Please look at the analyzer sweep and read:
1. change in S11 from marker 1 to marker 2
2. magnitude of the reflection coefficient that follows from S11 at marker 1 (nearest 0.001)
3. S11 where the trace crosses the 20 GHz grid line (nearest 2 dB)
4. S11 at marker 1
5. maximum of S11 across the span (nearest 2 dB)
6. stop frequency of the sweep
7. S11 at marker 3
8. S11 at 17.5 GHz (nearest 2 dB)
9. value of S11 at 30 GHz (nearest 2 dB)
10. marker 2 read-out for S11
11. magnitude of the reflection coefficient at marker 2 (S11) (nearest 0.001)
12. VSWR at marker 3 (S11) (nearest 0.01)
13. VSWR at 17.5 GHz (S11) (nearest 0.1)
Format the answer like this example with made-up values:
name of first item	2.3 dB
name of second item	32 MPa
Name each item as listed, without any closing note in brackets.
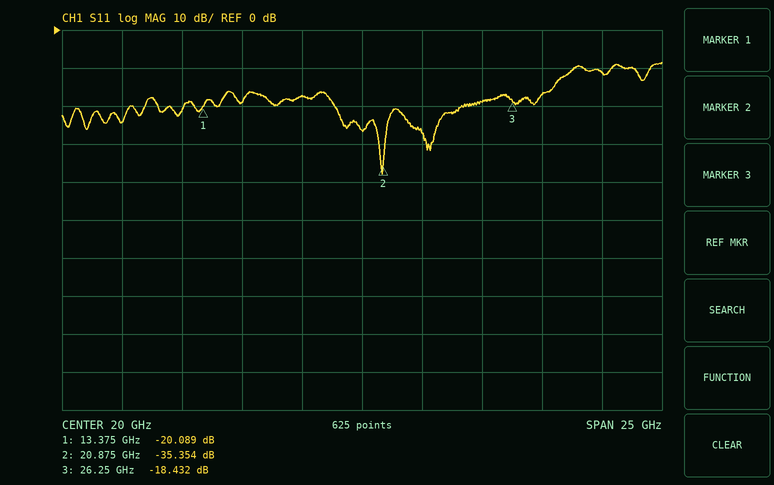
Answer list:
change in S11 from marker 1 to marker 2	-15.265 dB
magnitude of the reflection coefficient that follows from S11 at marker 1	0.099
S11 where the trace crosses the 20 GHz grid line	-26 dB
S11 at marker 1	-20.089 dB
maximum of S11 across the span	-8 dB
stop frequency of the sweep	32.5 GHz
S11 at marker 3	-18.432 dB
S11 at 17.5 GHz	-18 dB
value of S11 at 30 GHz	-12 dB
marker 2 read-out for S11	-35.354 dB
magnitude of the reflection coefficient at marker 2 (S11)	0.017
VSWR at marker 3 (S11)	1.27
VSWR at 17.5 GHz (S11)	1.3
